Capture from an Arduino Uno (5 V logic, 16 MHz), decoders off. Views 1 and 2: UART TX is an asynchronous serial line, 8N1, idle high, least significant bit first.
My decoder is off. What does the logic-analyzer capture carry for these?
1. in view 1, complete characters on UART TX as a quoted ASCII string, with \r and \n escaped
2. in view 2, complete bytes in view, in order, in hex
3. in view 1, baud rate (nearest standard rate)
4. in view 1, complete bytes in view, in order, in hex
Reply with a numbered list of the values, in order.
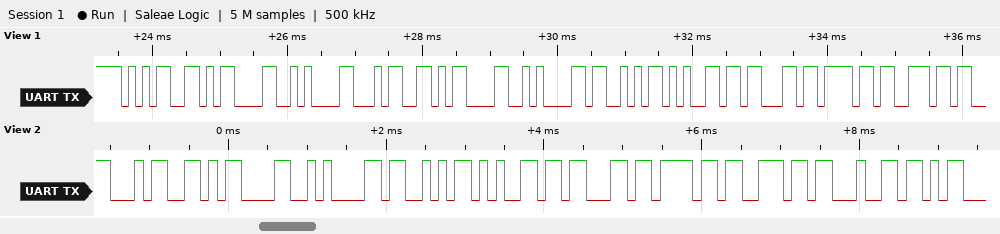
1. "5\r\n4\r\nSecon"
2. 34 0D 0A 53 65 63 6F 6E 64
3. 9600 baud
4. 35 0D 0A 34 0D 0A 53 65 63 6F 6E
